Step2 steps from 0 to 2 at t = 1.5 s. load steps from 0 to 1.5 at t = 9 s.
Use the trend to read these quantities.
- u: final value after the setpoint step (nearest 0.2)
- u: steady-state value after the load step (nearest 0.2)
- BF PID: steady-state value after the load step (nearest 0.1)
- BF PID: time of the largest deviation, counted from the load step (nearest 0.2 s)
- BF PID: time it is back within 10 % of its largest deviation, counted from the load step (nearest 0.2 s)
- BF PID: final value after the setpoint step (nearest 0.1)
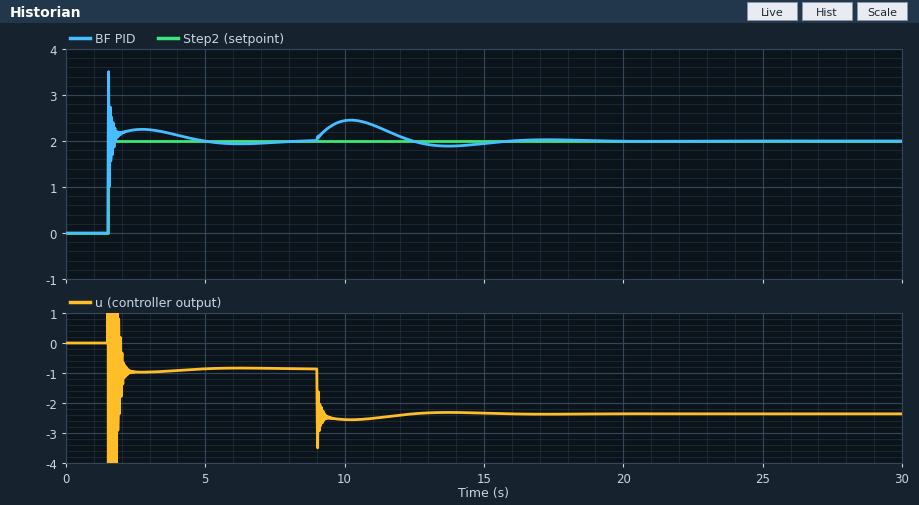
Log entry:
-0.8
-2.4
2.0
1.2 s
6.2 s
2.0
